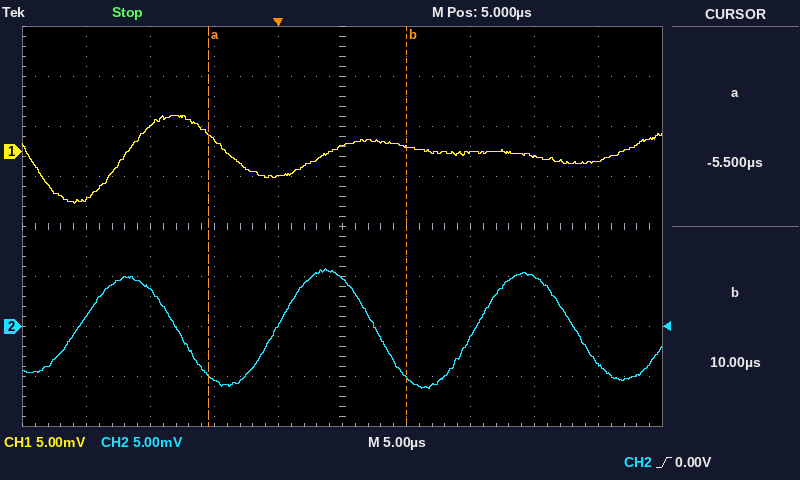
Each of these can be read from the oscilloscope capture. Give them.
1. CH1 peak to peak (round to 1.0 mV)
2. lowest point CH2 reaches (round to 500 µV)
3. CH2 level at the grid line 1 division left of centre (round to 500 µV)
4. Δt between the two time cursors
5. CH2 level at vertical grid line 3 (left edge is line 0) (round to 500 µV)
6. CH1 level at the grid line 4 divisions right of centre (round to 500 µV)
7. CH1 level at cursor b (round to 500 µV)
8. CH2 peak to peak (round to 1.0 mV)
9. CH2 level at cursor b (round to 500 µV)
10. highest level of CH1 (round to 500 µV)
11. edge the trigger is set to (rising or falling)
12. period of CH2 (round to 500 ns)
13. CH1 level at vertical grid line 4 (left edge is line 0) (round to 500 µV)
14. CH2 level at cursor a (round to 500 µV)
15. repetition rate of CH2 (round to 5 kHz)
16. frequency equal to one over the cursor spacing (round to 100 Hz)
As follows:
9.0 mV
-6.0 mV
0.0 mV
15.5 µs
-5.5 mV
-1.0 mV
500 µV
12.0 mV
-5.0 mV
3.5 mV
rising
15.5 µs
-2.5 mV
-5.0 mV
65 kHz
64.5 kHz
